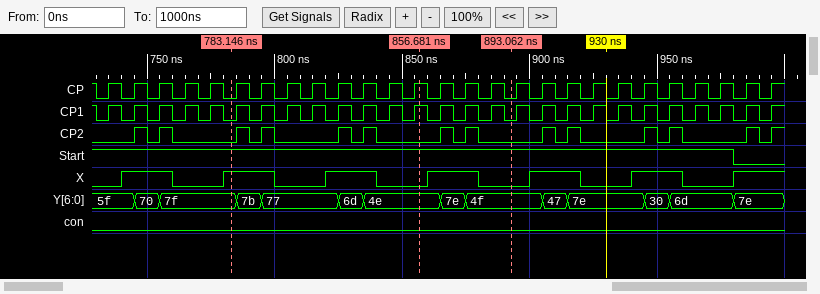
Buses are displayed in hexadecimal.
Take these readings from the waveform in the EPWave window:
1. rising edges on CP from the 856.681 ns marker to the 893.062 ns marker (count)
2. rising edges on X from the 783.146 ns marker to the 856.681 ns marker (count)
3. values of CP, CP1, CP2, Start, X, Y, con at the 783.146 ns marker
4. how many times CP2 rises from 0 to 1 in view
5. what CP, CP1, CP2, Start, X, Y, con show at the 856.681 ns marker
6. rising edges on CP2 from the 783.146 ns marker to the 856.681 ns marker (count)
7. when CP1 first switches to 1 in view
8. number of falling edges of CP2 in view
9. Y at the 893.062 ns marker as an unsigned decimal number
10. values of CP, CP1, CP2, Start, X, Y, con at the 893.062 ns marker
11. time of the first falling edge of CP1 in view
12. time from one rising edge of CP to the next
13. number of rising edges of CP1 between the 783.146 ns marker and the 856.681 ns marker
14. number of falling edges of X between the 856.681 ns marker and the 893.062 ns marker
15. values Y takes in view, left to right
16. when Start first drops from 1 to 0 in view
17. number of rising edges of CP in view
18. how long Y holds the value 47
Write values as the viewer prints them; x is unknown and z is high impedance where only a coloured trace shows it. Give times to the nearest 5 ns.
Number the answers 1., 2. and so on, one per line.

1. 3
2. 1
3. CP=0, CP1=0, CP2=0, Start=1, X=1, Y=7f, con=0
4. 14
5. CP=1, CP1=1, CP2=0, Start=1, X=0, Y=4e, con=0
6. 4
7. 735 ns
8. 13
9. 79
10. CP=0, CP1=0, CP2=0, Start=1, X=0, Y=4f, con=0
11. 730 ns
12. 10 ns
13. 8
14. 1
15. 5f, 70, 7f, 7b, 77, 6d, 4e, 7e, 4f, 47, 7e, 30, 6d, 7e
16. 980 ns
17. 27
18. 10 ns
